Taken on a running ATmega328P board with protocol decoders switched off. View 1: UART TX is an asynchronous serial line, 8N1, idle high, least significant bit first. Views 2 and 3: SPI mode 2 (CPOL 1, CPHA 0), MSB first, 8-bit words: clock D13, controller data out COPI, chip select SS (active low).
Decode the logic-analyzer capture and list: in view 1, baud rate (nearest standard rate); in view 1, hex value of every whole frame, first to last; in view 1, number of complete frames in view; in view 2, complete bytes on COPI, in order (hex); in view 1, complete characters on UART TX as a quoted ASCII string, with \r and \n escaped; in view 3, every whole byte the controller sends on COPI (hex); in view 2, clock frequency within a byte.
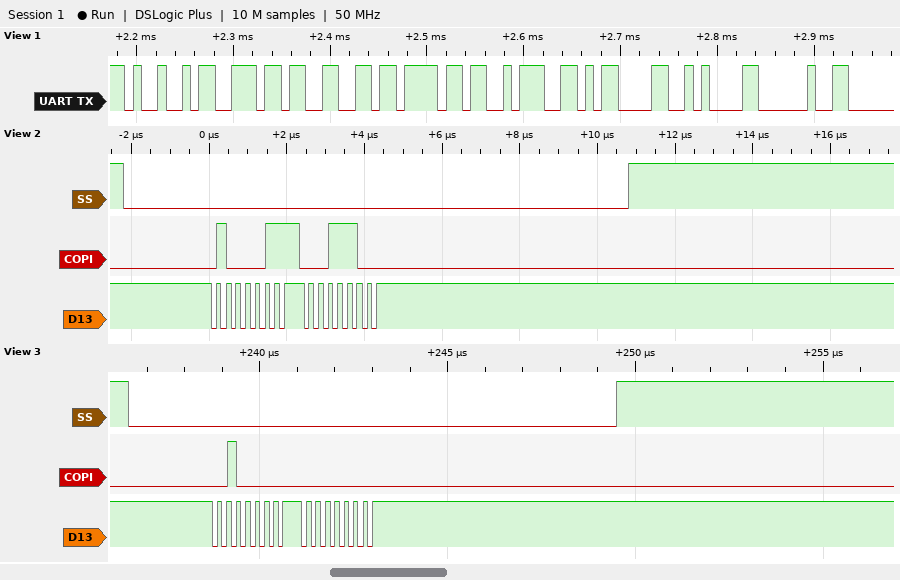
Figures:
115200 baud
49 6E 66 6F 3A 0D 0A 20
8
43 1C
"Info:\r\n "
0x20 0x00
4 MHz
